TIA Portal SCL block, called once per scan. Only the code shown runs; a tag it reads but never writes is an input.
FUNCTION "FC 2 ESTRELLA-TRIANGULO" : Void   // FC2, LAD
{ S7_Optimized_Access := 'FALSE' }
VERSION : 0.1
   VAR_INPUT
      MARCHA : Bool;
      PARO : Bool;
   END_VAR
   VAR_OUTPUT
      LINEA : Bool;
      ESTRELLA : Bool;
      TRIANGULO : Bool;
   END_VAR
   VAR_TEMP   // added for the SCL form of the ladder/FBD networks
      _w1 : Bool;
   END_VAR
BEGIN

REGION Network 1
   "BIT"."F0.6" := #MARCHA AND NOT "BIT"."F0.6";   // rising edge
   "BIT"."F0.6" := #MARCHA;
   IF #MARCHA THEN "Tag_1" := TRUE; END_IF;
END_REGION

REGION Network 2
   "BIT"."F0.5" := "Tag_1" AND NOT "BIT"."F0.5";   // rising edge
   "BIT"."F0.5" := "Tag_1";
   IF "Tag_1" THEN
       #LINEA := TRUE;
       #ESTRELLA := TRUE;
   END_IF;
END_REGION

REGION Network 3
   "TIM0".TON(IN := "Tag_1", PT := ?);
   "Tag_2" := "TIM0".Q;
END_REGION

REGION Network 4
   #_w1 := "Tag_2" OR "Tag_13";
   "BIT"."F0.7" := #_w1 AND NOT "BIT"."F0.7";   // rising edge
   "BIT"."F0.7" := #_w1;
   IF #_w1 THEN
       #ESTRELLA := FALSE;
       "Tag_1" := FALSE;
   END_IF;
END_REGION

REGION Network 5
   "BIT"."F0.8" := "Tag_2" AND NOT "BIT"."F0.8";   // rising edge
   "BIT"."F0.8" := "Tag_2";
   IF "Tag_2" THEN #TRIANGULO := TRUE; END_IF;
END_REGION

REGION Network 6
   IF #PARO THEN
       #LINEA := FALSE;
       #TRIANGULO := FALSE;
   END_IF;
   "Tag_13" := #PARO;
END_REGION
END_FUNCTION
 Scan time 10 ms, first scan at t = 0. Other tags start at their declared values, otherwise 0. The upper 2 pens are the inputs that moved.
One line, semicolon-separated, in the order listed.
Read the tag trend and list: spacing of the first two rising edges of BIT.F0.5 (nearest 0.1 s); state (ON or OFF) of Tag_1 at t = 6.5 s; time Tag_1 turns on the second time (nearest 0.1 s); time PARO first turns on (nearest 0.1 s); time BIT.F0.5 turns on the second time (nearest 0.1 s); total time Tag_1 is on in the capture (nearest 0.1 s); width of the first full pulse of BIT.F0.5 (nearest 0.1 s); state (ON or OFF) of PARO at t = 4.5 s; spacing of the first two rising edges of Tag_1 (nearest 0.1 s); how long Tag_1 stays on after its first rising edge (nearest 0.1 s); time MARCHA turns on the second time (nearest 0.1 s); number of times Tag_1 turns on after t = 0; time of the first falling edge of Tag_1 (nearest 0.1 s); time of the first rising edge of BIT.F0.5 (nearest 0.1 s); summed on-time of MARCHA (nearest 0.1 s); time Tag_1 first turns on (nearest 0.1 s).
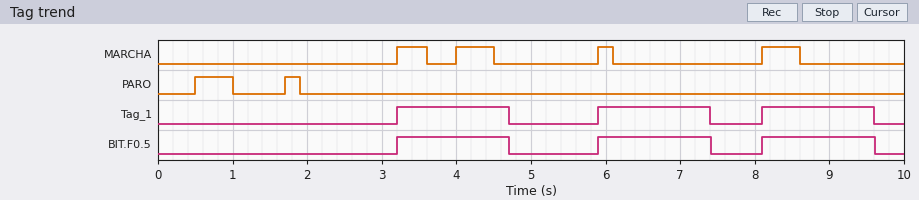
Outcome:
2.7 s; ON; 5.9 s; 0.5 s; 5.9 s; 4.5 s; 1.5 s; OFF; 2.7 s; 1.5 s; 4.0 s; 3; 4.7 s; 3.2 s; 1.6 s; 3.2 s
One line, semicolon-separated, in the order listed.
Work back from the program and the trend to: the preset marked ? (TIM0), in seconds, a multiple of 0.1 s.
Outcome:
1.5 s
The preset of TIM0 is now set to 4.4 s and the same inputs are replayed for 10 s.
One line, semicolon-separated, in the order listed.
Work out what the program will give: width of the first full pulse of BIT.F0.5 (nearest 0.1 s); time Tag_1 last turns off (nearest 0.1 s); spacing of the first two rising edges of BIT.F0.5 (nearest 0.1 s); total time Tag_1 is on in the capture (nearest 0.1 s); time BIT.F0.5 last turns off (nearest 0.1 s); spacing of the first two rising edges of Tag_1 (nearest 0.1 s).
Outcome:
4.4 s; 7.6 s; 4.9 s; 6.3 s; 7.6 s; 4.9 s
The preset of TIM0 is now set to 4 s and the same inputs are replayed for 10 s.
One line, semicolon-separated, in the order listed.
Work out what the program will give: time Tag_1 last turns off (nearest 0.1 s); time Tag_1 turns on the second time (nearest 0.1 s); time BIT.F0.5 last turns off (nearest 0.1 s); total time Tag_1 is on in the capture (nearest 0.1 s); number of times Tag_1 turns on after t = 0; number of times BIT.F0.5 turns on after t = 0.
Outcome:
7.2 s; 8.1 s; 7.2 s; 5.9 s; 2; 2
